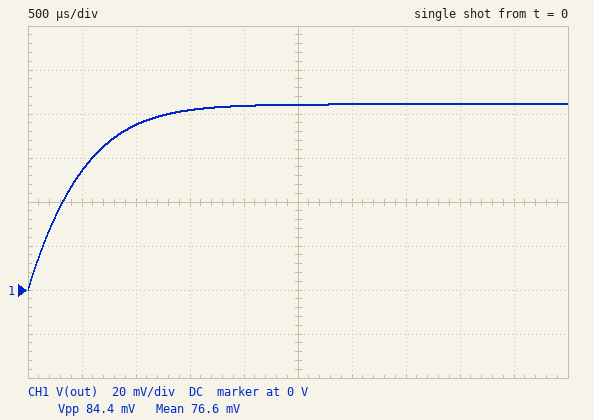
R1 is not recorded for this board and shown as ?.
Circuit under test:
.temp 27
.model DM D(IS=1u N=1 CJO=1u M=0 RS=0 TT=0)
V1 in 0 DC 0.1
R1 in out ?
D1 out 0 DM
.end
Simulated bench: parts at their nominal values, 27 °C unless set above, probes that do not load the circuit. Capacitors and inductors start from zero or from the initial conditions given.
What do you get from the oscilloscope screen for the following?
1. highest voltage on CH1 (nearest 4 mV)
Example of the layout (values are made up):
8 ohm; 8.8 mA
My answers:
84 mV
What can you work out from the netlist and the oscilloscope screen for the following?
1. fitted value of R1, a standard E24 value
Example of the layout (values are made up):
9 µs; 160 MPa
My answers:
620 Ω
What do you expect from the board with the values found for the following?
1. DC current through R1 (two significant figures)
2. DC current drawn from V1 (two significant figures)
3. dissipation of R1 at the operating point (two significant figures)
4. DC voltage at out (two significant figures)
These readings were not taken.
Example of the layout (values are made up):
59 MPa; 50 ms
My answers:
25 µA; 25 µA; 390 nW; 84 mV
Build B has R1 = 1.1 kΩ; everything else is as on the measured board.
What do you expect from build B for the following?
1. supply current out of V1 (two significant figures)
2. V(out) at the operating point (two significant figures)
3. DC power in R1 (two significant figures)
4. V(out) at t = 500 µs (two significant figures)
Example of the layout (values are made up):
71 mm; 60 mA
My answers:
20 µA; 78 mV; 430 nW; 36 mV
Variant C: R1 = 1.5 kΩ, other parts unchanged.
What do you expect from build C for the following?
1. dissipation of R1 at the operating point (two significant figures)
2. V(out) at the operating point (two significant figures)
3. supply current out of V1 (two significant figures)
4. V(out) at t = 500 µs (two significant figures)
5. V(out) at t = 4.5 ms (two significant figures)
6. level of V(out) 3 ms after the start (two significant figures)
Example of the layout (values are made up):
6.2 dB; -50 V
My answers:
430 nW; 75 mV; 17 µA; 28 mV; 74 mV; 72 mV
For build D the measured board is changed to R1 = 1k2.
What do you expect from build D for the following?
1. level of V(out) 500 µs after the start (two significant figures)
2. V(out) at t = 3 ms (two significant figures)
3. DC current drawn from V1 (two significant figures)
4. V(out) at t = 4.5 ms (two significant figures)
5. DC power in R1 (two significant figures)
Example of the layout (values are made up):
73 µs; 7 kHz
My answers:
34 mV; 76 mV; 19 µA; 77 mV; 430 nW
